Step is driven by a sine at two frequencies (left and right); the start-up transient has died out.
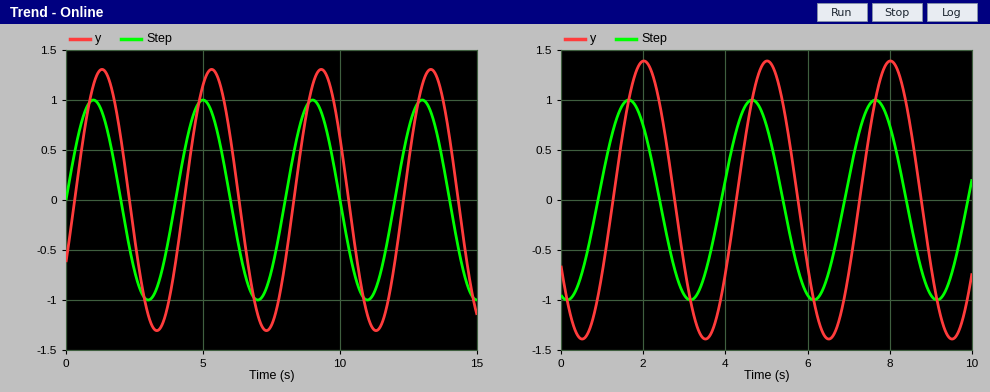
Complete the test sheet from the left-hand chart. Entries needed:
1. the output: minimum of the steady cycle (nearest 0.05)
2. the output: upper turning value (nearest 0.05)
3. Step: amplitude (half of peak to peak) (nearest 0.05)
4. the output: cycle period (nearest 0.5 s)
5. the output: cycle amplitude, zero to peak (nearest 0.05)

-1.30
1.30
1.00
4.0 s
1.30
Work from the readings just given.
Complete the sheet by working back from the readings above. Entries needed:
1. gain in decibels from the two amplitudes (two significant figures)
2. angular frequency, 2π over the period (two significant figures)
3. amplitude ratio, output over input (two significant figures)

2.3 dB
1.6 rad/s
1.3
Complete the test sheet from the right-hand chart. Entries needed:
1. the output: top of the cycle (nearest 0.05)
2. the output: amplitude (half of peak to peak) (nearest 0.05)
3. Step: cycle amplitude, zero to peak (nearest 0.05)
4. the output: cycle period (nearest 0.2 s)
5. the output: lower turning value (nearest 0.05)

1.40
1.40
1.00
3.0 s
-1.40
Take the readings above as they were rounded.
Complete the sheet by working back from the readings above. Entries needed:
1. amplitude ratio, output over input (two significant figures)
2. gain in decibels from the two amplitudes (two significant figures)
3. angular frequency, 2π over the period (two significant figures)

1.4
2.9 dB
2.1 rad/s
